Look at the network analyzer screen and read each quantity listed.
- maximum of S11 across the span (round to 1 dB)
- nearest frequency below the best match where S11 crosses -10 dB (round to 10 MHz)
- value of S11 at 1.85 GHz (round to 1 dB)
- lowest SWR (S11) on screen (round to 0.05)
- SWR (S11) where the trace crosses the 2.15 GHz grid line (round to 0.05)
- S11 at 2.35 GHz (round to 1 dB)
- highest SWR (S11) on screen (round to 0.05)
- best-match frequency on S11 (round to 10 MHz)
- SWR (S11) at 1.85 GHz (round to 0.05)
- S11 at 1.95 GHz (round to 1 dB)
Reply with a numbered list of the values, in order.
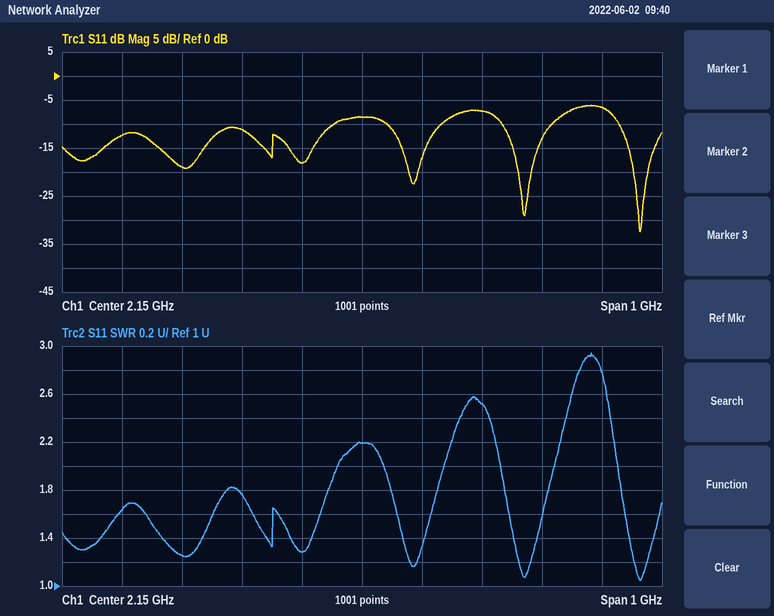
1. -6 dB
2. 2.58 GHz
3. -19 dB
4. 1.05
5. 2.20
6. -7 dB
7. 2.95
8. 2.61 GHz
9. 1.25
10. -11 dB
